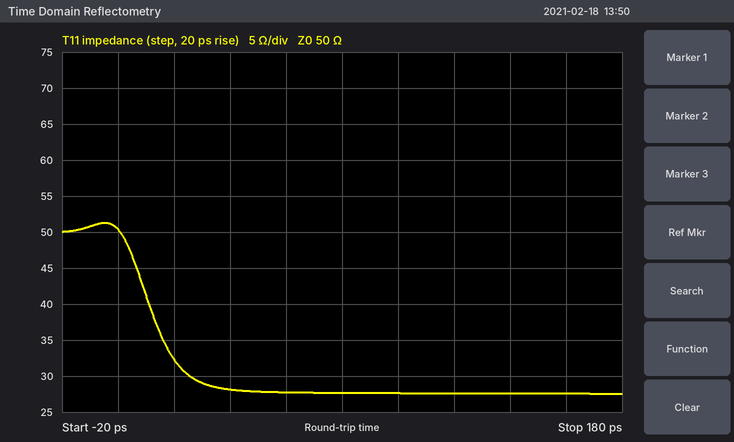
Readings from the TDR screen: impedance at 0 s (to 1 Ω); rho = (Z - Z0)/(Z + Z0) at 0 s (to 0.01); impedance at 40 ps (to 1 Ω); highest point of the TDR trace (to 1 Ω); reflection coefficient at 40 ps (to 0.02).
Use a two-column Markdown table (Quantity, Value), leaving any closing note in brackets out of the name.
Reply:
| Quantity | Value |
|---|---|
| impedance at 0 s | 50 Ω |
| rho = (Z - Z0)/(Z + Z0) at 0 s | 0.00 |
| impedance at 40 ps | 28 Ω |
| highest point of the TDR trace | 51 Ω |
| reflection coefficient at 40 ps | -0.28 |
